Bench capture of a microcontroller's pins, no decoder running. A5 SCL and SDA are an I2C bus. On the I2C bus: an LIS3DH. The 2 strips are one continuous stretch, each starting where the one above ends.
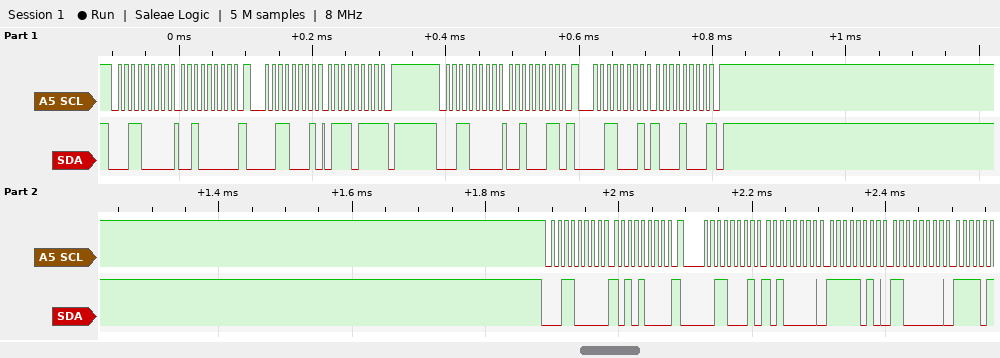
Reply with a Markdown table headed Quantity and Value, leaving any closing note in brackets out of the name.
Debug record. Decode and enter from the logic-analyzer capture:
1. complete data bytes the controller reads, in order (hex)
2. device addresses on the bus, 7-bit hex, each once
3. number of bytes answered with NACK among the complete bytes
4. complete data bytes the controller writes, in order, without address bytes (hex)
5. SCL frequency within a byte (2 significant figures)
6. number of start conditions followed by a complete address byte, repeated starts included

| Quantity | Value |
|---|---|
| complete data bytes the controller reads, in order | 77 88 A0 FA C0 |
| device addresses on the bus, 7-bit hex, each once | 0x18 |
| number of bytes answered with NACK among the complete bytes | 2 |
| complete data bytes the controller writes, in order, without address bytes | 20 23 A8 |
| SCL frequency within a byte | 100 kHz |
| number of start conditions followed by a complete address byte, repeated starts included | 6 |
